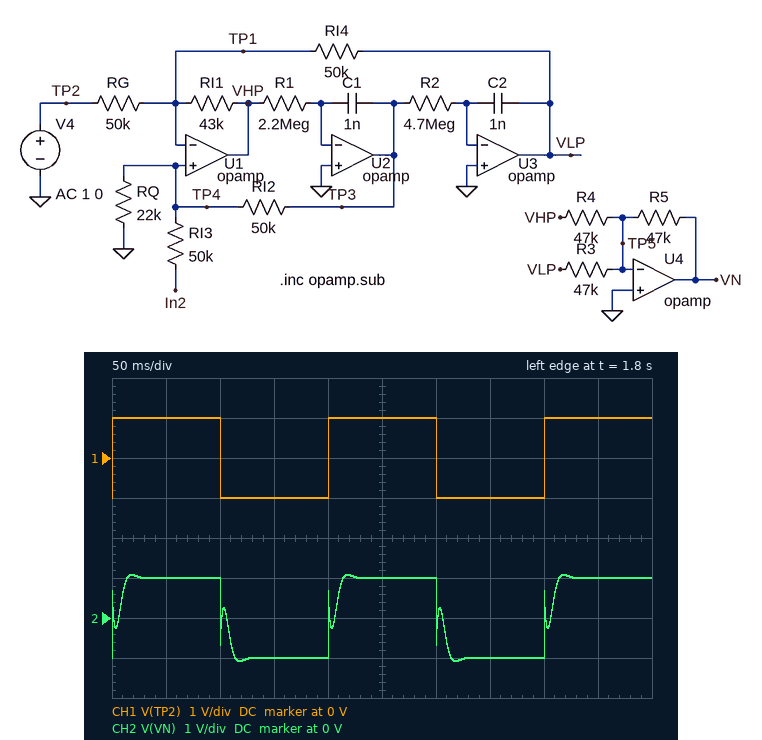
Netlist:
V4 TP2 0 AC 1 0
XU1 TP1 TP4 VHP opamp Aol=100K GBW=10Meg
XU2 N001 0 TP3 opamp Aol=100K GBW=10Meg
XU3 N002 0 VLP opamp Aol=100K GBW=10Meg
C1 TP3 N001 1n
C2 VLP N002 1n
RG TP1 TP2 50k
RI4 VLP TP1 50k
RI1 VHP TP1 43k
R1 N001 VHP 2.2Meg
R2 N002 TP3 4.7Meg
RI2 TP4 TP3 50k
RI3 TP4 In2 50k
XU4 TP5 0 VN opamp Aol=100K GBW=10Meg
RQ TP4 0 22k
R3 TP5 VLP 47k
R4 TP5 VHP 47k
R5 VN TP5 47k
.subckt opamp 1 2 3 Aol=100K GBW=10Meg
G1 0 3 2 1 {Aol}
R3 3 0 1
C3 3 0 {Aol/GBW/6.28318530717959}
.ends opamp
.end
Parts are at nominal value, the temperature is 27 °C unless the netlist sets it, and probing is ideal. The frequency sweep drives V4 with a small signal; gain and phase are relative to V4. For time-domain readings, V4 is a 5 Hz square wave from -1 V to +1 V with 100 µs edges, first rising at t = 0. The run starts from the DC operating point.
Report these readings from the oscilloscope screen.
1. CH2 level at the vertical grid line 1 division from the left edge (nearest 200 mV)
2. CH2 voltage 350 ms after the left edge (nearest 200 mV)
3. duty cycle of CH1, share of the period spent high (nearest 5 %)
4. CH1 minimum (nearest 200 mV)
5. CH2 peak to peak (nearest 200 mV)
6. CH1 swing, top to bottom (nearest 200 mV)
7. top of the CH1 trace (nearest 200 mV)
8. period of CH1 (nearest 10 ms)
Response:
1.0 V
-1.0 V
50 %
-1.0 V
2.2 V
2.0 V
1.0 V
200 ms
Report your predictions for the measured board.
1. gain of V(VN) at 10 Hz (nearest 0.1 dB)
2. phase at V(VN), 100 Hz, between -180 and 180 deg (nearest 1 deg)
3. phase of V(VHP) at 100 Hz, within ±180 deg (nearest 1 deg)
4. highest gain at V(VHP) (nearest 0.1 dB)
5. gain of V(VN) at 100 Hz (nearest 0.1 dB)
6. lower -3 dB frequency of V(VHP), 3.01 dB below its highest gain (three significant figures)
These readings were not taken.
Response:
-0.3 dB
37 deg
-143 deg
-1.2 dB
-3.7 dB
43.1 Hz
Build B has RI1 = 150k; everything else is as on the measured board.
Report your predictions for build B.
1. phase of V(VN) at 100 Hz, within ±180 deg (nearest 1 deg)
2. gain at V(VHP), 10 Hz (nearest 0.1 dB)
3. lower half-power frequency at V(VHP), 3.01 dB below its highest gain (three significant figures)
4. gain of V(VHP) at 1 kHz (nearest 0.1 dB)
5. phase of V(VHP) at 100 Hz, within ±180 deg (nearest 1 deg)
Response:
80 deg
-27.9 dB
115 Hz
9.5 dB
-100 deg
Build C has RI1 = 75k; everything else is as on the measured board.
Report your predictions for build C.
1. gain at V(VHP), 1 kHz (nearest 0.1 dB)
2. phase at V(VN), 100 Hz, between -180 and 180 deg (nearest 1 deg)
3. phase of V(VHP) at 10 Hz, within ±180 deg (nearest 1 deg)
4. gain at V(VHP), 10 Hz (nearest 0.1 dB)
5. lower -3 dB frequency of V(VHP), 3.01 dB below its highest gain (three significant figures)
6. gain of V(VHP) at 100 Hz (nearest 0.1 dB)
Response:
3.5 dB
54 deg
-14 deg
-27.8 dB
62.6 Hz
2.8 dB
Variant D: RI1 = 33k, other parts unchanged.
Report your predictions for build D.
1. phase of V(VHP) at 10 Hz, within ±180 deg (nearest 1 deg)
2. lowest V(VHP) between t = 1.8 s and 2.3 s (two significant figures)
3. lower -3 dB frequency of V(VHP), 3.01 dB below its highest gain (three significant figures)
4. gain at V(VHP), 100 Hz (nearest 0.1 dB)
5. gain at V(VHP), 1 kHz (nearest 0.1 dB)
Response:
-19 deg
-1.3 V
37.2 Hz
-3.5 dB
-3.6 dB
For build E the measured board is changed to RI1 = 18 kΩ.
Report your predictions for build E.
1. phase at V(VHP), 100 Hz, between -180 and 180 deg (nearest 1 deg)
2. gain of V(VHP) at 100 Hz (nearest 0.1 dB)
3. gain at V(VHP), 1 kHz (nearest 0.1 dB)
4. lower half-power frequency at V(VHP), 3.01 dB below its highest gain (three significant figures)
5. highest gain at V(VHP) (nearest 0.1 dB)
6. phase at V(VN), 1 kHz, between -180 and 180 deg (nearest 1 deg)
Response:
-157 deg
-8.8 dB
-8.9 dB
27.5 Hz
-8.7 dB
2 deg
